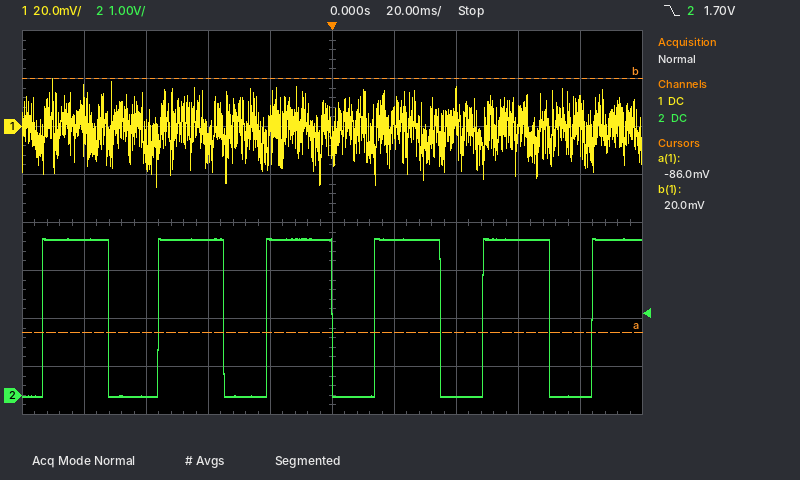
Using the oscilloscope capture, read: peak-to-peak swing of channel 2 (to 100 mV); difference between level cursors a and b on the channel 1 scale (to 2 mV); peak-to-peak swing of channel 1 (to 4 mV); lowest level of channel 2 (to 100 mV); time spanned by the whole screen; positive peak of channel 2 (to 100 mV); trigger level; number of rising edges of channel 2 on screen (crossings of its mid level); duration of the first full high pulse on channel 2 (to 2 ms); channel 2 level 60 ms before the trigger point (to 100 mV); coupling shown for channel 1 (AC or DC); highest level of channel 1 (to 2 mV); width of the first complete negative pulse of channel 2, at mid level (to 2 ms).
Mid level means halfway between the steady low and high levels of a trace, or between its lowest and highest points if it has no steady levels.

3.3 V
106 mV
44 mV
0.0 V
200 ms
3.3 V
1.70 V
6
22 ms
0.0 V
DC
20 mV
16 ms
